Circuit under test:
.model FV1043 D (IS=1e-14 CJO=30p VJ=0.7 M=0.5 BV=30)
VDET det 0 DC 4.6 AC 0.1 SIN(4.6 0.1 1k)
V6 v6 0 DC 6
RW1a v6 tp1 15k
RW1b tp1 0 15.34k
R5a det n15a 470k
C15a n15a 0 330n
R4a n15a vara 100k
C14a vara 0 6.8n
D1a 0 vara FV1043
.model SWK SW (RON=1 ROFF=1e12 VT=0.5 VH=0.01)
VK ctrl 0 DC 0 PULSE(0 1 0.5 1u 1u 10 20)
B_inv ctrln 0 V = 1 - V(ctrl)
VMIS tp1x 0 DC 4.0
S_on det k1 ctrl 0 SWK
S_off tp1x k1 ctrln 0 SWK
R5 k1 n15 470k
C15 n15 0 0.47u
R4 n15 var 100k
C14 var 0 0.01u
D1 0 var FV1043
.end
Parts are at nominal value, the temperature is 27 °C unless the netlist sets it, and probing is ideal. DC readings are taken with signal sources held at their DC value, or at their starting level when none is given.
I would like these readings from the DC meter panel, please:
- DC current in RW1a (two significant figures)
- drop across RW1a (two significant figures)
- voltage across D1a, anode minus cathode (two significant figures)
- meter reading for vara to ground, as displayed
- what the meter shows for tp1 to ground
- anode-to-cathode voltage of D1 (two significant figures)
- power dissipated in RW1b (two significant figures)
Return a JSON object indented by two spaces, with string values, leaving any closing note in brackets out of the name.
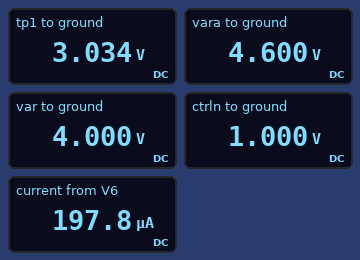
{
  "DC current in RW1a": "200 µA",
  "drop across RW1a": "3.0 V",
  "voltage across D1a, anode minus cathode": "-4.6 V",
  "meter reading for vara to ground, as displayed": "4.600 V",
  "what the meter shows for tp1 to ground": "3.034 V",
  "anode-to-cathode voltage of D1": "-4.0 V",
  "power dissipated in RW1b": "600 µW"
}
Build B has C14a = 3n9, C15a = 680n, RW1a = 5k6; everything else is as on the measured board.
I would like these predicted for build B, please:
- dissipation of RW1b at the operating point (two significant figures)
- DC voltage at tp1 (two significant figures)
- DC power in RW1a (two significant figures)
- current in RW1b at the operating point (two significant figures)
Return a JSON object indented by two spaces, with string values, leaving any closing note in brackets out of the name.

{
  "dissipation of RW1b at the operating point": "1.3 mW",
  "DC voltage at tp1": "4.4 V",
  "DC power in RW1a": "460 µW",
  "current in RW1b at the operating point": "290 µA"
}
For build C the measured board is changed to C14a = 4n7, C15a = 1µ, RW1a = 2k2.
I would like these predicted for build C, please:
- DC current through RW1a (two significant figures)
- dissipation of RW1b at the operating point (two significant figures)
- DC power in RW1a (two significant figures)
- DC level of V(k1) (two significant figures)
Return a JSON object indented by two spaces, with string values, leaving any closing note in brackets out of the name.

{
  "DC current through RW1a": "340 µA",
  "dissipation of RW1b at the operating point": "1.8 mW",
  "DC power in RW1a": "260 µW",
  "DC level of V(k1)": "4.0 V"
}
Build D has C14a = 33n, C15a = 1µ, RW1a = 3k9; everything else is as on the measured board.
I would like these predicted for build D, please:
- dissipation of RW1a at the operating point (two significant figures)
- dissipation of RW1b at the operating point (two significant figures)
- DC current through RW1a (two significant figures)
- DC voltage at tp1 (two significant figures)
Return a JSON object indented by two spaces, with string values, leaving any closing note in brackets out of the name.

{
  "dissipation of RW1a at the operating point": "380 µW",
  "dissipation of RW1b at the operating point": "1.5 mW",
  "DC current through RW1a": "310 µA",
  "DC voltage at tp1": "4.8 V"
}
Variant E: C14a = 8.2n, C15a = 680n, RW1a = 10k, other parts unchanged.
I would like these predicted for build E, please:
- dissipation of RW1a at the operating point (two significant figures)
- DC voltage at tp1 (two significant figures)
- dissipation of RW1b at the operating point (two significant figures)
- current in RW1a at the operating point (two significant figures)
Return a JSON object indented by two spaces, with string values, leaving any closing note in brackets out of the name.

{
  "dissipation of RW1a at the operating point": "560 µW",
  "DC voltage at tp1": "3.6 V",
  "dissipation of RW1b at the operating point": "860 µW",
  "current in RW1a at the operating point": "240 µA"
}
